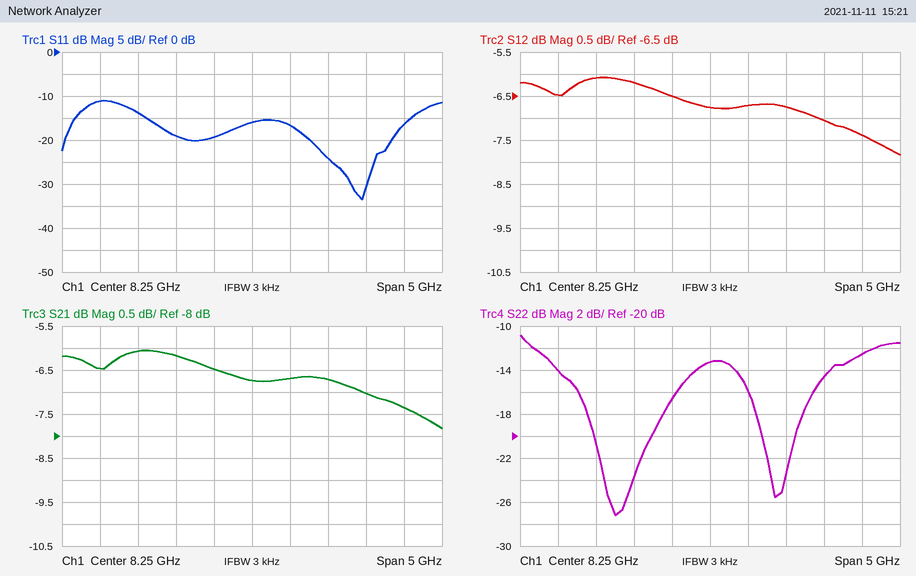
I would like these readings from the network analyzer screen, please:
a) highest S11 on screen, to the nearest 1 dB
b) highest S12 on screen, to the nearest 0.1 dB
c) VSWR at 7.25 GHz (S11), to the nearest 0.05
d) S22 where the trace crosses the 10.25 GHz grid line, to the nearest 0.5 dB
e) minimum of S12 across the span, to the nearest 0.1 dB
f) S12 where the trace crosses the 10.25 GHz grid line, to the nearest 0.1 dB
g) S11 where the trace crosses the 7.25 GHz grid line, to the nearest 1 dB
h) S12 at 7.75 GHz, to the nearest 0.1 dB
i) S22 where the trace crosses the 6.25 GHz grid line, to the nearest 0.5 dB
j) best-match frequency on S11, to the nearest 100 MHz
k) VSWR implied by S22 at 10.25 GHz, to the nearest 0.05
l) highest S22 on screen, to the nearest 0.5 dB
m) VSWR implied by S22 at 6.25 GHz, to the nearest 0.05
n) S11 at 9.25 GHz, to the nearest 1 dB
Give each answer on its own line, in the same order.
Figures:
-11 dB
-6.1 dB
1.25
-12.5 dB
-7.8 dB
-7.4 dB
-19 dB
-6.5 dB
-14.0 dB
9.7 GHz
1.60
-11.0 dB
1.50
-24 dB
